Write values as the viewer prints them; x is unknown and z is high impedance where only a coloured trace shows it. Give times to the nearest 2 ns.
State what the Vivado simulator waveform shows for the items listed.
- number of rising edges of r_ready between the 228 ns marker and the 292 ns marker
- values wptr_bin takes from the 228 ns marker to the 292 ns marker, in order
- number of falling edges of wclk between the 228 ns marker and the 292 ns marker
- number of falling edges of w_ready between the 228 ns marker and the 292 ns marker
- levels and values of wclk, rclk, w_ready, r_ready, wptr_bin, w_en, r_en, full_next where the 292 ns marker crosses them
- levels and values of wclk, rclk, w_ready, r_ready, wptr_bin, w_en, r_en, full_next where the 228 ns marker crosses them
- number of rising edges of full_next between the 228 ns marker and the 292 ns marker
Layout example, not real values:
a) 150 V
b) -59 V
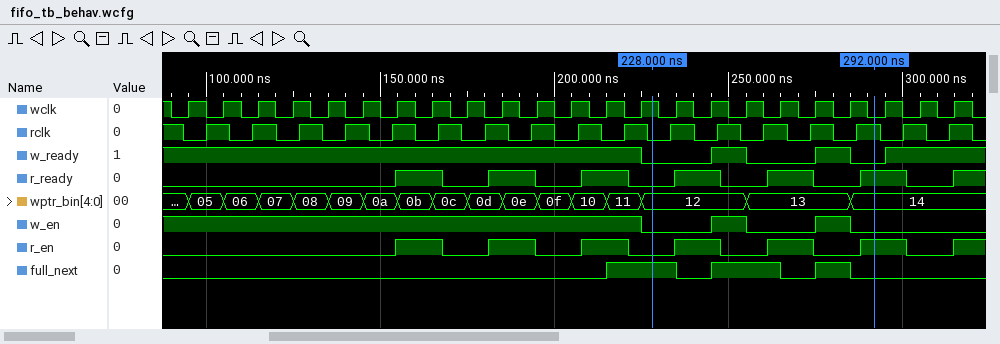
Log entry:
a) 3
b) 12, 13, 14
c) 7
d) 2
e) wclk=0, rclk=1, w_ready=0, r_ready=1, wptr_bin=14, w_en=0, r_en=1, full_next=0
f) wclk=1, rclk=0, w_ready=0, r_ready=0, wptr_bin=12, w_en=0, r_en=0, full_next=1
g) 2
